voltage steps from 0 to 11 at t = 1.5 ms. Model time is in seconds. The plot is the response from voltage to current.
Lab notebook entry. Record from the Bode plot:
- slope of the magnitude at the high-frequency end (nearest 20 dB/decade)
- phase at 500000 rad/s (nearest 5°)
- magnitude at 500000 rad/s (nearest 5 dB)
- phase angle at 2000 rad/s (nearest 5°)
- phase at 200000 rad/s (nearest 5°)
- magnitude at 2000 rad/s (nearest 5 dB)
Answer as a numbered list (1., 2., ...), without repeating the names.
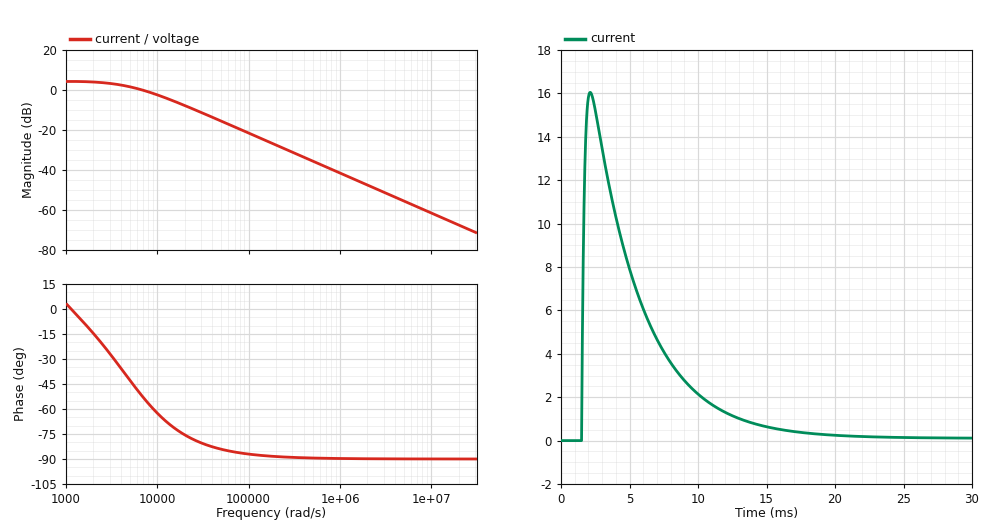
1. -20 dB/decade
2. -90°
3. -35 dB
4. -15°
5. -90°
6. 5 dB
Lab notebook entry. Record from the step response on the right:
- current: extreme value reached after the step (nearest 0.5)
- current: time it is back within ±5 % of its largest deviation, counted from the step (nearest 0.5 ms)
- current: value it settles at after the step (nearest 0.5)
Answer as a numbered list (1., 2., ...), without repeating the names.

1. 16.0
2. 12.0 ms
3. 0.0
